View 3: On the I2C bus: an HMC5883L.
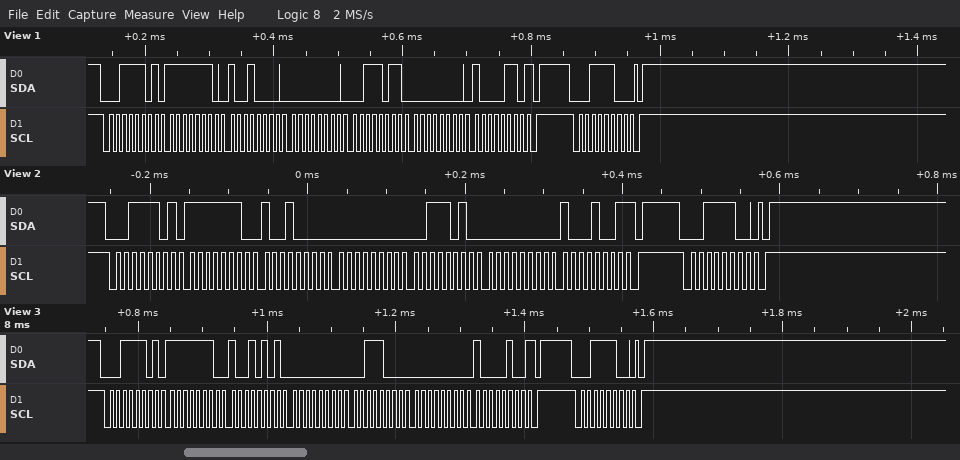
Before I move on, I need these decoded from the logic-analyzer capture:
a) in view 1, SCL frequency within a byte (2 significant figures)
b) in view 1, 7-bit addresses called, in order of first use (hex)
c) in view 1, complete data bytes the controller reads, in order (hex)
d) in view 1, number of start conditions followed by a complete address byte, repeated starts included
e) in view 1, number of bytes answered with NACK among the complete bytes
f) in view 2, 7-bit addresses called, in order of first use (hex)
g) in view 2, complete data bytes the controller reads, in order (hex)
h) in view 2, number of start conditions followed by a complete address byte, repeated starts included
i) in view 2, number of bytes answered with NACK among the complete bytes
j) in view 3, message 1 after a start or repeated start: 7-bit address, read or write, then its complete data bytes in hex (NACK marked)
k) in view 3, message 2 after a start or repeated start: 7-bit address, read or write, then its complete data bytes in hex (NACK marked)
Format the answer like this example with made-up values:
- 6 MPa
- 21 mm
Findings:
- 100 kHz
- 0x1E
- FE 90 00 3B 00 86
- 2
- 1
- 0x1E
- FE 90 00 3A 00 89
- 2
- 1
- 0x1E read: FE 95 00 38 00 84 NACK
- 0x1E write
